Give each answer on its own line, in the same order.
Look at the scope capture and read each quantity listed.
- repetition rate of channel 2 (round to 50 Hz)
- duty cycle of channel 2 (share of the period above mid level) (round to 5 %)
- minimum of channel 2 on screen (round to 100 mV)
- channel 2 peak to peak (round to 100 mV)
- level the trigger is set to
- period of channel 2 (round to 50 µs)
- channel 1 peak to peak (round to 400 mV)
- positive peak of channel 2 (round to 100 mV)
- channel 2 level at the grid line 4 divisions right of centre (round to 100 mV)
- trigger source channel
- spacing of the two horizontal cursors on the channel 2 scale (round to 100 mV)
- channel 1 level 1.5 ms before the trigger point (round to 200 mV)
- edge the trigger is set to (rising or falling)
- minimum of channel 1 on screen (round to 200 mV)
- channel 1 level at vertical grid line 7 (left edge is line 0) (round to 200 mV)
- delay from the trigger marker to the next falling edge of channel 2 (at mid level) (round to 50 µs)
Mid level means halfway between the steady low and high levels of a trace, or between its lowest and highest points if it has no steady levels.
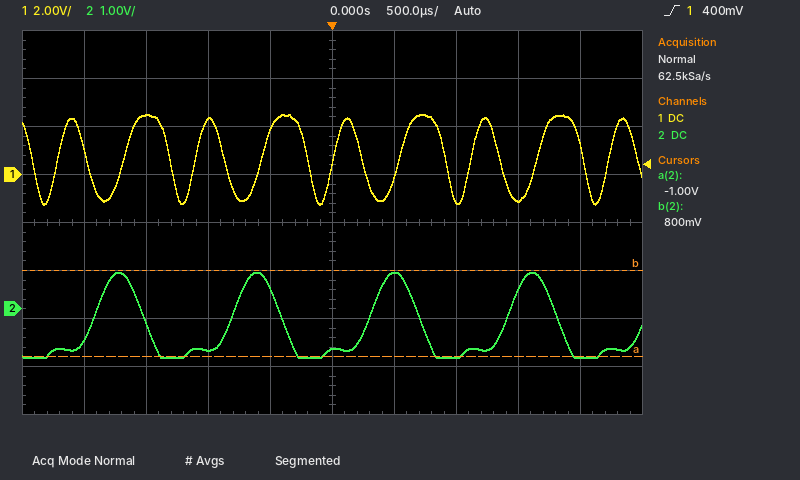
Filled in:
900 Hz
35 %
-1.0 V
1.8 V
400 mV
1.10 ms
3.6 V
800 mV
-1.0 V
channel 1
1.8 V
2.4 V
rising
-1.2 V
-1.0 V
700 µs
